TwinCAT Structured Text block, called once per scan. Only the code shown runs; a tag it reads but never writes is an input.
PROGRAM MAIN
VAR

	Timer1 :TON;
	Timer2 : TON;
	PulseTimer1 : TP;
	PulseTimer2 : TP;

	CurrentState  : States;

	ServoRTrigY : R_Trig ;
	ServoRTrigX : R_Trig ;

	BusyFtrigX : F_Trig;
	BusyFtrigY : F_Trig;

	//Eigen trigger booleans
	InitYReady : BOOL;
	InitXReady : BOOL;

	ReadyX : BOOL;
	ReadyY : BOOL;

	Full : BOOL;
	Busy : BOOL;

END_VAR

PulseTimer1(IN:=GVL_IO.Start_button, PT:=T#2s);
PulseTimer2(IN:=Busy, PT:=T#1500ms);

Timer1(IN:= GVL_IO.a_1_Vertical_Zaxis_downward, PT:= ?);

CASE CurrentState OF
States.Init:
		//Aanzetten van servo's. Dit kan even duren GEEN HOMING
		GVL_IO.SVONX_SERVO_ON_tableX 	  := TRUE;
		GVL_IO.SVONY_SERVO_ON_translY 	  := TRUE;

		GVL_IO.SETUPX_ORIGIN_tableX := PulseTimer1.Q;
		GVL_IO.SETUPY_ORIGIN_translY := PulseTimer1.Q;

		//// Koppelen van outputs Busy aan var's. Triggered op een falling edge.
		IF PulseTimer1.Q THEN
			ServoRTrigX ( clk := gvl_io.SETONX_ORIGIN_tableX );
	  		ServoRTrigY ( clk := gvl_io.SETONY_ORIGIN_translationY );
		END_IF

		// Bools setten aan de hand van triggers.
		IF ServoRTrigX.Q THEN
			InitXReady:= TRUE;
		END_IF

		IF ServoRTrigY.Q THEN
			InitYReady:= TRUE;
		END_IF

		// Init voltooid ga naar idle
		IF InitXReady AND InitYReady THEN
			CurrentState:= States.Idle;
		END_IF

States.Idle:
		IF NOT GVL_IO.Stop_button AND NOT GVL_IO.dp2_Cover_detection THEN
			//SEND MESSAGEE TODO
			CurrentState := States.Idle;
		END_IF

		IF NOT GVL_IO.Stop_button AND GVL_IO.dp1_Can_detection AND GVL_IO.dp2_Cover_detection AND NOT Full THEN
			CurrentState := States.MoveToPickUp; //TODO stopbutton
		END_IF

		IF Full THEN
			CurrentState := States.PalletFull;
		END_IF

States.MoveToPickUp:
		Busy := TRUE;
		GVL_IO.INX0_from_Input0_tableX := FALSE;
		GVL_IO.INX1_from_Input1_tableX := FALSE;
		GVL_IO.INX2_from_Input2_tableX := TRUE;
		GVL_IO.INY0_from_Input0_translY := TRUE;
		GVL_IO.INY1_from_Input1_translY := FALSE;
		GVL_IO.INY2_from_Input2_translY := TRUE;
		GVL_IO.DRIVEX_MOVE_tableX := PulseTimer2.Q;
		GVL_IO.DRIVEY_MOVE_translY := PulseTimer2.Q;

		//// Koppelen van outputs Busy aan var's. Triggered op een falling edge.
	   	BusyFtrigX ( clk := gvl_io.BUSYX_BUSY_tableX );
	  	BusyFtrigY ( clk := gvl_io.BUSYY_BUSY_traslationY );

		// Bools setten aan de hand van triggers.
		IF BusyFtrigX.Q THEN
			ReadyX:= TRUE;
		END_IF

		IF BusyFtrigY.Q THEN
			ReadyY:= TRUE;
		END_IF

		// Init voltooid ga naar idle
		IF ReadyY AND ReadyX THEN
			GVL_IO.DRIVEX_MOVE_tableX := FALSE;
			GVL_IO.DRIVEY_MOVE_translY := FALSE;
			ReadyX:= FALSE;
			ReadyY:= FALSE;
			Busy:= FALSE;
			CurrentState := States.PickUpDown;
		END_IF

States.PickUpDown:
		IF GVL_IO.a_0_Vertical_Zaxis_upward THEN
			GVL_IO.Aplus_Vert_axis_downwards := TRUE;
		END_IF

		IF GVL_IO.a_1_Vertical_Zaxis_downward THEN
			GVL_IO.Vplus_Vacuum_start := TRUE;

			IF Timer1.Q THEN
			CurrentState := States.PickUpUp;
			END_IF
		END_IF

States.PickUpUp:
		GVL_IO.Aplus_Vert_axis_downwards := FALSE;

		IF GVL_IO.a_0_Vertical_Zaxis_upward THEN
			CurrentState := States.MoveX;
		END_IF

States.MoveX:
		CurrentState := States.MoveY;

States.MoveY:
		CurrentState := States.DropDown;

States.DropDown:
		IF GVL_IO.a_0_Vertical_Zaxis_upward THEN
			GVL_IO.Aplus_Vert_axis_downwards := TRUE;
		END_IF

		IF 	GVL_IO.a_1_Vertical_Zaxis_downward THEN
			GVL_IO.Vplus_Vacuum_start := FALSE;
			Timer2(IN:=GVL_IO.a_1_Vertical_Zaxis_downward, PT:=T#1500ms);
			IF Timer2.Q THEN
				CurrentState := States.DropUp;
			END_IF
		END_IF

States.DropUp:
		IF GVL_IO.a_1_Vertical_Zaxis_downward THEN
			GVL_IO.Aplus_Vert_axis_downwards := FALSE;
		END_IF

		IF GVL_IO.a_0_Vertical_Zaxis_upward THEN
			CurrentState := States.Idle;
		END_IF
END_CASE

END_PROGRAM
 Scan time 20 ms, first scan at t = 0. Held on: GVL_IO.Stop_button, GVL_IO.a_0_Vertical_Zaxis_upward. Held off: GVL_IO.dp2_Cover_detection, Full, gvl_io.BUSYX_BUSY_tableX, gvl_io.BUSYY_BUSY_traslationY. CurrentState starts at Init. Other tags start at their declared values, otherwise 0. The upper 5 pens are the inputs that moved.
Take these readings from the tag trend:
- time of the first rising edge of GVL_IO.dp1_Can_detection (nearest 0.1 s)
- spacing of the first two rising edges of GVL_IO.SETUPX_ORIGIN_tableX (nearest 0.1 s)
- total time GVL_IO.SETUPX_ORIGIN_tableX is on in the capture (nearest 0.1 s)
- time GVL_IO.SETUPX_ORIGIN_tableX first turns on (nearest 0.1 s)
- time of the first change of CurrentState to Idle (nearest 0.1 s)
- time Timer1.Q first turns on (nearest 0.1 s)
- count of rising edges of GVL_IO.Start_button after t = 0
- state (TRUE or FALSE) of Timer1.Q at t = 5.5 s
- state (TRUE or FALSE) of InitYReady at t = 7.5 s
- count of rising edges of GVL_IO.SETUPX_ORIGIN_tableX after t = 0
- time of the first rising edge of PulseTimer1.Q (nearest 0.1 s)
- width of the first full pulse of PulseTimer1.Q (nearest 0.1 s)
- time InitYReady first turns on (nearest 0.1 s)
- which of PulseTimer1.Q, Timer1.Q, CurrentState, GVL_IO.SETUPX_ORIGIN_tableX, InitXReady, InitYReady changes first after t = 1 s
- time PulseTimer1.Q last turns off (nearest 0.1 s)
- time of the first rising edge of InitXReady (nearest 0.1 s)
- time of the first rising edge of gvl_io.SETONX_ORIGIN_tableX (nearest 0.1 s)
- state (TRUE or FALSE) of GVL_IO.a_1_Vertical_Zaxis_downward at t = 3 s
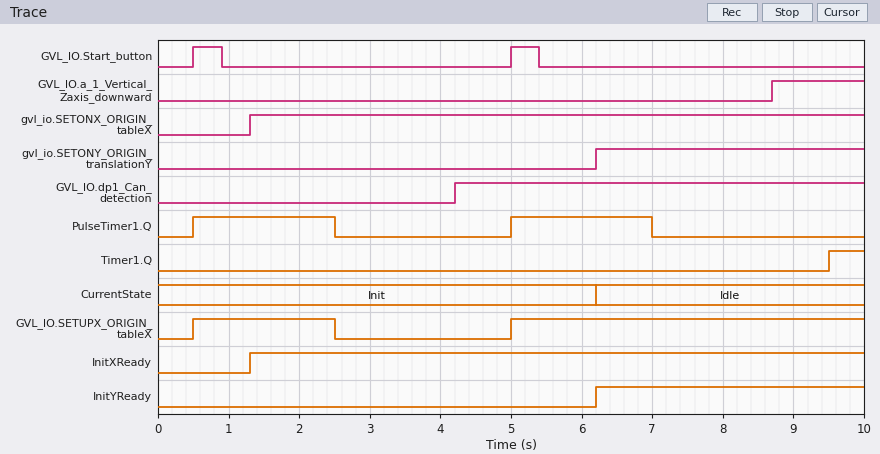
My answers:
4.2 s
4.5 s
7.0 s
0.5 s
6.2 s
9.5 s
2
FALSE
TRUE
2
0.5 s
2.0 s
6.2 s
InitXReady
7.0 s
1.3 s
1.3 s
FALSE
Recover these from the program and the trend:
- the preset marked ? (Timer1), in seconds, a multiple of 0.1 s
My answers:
0.8 s
